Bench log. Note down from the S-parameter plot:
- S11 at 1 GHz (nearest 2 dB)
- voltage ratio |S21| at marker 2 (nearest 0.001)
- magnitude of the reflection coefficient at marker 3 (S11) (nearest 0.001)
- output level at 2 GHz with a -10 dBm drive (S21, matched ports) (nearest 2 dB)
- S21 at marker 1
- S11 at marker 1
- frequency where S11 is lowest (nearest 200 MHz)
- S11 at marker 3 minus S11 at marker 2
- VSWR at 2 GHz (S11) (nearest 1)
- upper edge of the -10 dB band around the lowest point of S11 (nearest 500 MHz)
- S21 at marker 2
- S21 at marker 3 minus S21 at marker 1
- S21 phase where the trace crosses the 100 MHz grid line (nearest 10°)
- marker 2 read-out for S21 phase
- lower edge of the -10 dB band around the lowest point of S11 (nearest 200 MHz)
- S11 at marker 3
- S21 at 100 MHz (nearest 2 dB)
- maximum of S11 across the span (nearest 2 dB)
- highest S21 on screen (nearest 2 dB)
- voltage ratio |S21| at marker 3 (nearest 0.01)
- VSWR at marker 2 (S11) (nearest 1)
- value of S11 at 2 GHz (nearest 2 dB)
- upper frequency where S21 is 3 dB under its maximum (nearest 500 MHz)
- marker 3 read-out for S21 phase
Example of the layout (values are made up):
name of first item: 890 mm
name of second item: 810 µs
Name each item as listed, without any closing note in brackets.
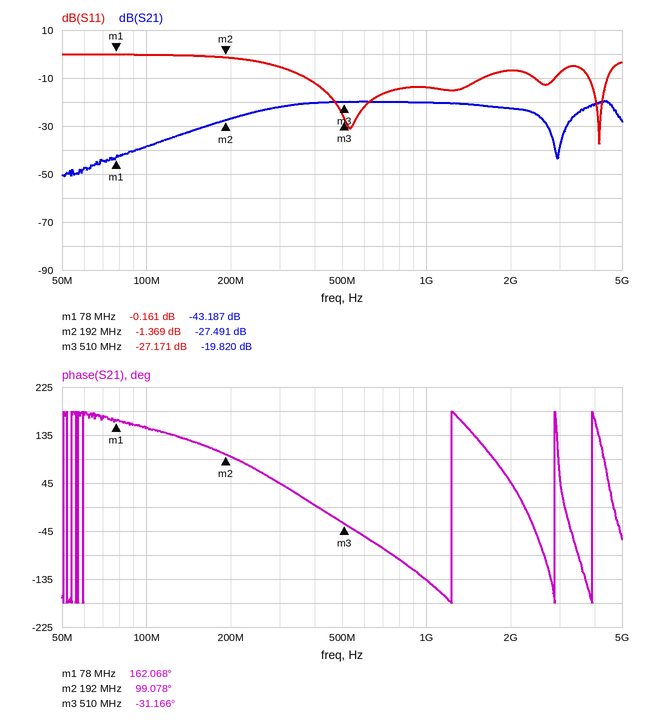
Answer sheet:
S11 at 1 GHz: -14 dB
voltage ratio |S21| at marker 2: 0.042
magnitude of the reflection coefficient at marker 3 (S11): 0.044
output level at 2 GHz with a -10 dBm drive (S21, matched ports): -32 dBm
S21 at marker 1: -43.187 dB
S11 at marker 1: -0.161 dB
frequency where S11 is lowest: 4.2 GHz
S11 at marker 3 minus S11 at marker 2: -25.802 dB
VSWR at 2 GHz (S11): 3
upper edge of the -10 dB band around the lowest point of S11: 4.5 GHz
S21 at marker 2: -27.491 dB
S21 at marker 3 minus S21 at marker 1: 23.367 dB
S21 phase where the trace crosses the 100 MHz grid line: 150°
marker 2 read-out for S21 phase: 99.078°
lower edge of the -10 dB band around the lowest point of S11: 3.8 GHz
S11 at marker 3: -27.171 dB
S21 at 100 MHz: -38 dB
maximum of S11 across the span: 0 dB
highest S21 on screen: -20 dB
voltage ratio |S21| at marker 3: 0.10
VSWR at marker 2 (S11): 13
value of S11 at 2 GHz: -6 dB
upper frequency where S21 is 3 dB under its maximum: 4.5 GHz
marker 3 read-out for S21 phase: -31.166°
